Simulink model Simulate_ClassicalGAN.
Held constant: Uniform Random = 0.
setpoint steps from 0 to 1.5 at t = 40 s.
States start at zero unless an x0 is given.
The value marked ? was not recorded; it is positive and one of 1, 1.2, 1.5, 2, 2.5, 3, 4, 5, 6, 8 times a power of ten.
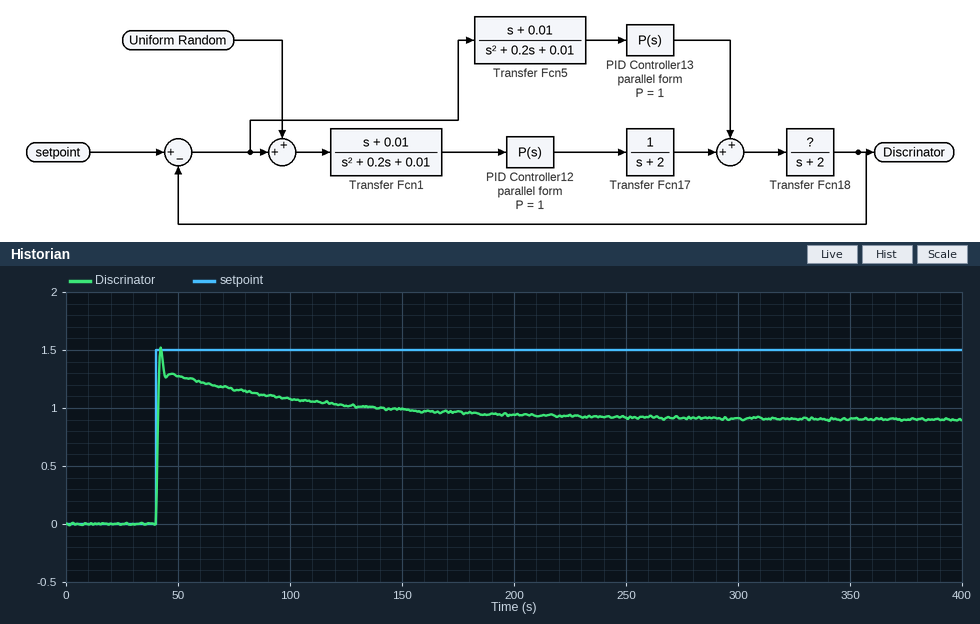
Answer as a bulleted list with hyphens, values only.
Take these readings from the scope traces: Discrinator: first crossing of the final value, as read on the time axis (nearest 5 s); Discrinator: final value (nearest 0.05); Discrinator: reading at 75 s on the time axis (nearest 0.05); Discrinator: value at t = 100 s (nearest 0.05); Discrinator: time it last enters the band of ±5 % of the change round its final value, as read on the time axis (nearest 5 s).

- 40 s
- 0.90
- 1.15
- 1.10
- 195 s
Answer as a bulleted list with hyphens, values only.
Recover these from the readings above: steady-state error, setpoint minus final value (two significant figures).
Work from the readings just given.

- 0.60
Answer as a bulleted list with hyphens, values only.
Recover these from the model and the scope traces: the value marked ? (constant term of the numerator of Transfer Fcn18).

- 2
